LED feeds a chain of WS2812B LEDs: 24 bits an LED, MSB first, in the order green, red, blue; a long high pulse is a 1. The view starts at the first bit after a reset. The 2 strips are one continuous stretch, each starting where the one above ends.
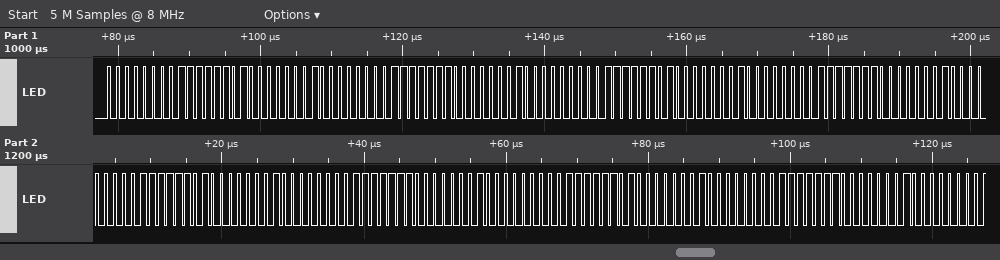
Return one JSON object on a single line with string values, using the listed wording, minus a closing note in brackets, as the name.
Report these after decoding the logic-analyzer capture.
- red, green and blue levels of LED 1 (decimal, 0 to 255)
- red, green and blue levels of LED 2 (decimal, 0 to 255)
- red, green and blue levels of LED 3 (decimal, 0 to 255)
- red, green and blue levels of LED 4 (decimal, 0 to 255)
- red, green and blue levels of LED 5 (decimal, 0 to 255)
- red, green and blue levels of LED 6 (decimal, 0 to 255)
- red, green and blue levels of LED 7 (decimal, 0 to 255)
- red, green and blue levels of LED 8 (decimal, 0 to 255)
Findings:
{"red, green and blue levels of LED 1": "253, 0, 1", "red, green and blue levels of LED 2": "254, 0, 2", "red, green and blue levels of LED 3": "253, 0, 1", "red, green and blue levels of LED 4": "254, 0, 2", "red, green and blue levels of LED 5": "253, 0, 1", "red, green and blue levels of LED 6": "254, 0, 2", "red, green and blue levels of LED 7": "253, 0, 1", "red, green and blue levels of LED 8": "254, 0, 2"}
